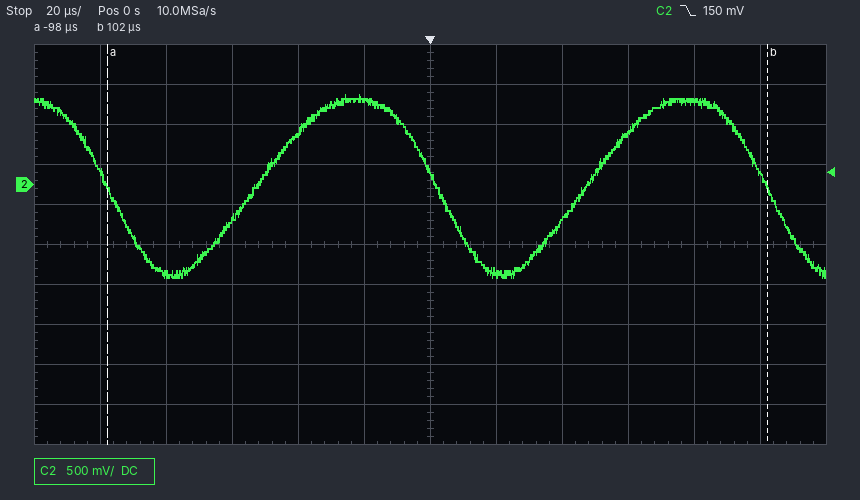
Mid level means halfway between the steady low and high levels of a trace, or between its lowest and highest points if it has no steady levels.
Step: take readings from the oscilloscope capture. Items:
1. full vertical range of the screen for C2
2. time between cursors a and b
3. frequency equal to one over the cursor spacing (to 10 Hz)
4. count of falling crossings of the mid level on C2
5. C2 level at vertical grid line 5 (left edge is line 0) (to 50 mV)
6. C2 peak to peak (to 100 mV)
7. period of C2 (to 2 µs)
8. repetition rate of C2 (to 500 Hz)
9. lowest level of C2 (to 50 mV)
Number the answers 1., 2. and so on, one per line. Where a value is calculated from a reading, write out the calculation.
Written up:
1. 5 V
2. 102 µs − (-98 µs) = 200 µs
3. 1 / 200 µs ≈ 5.00 kHz
4. 3
5. 1.05 V
6. 2.30 V
7. 100 µs
8. 1 / 100 µs ≈ 10.0 kHz
9. -1.15 V
